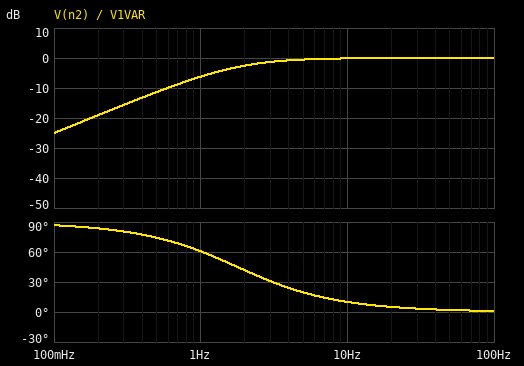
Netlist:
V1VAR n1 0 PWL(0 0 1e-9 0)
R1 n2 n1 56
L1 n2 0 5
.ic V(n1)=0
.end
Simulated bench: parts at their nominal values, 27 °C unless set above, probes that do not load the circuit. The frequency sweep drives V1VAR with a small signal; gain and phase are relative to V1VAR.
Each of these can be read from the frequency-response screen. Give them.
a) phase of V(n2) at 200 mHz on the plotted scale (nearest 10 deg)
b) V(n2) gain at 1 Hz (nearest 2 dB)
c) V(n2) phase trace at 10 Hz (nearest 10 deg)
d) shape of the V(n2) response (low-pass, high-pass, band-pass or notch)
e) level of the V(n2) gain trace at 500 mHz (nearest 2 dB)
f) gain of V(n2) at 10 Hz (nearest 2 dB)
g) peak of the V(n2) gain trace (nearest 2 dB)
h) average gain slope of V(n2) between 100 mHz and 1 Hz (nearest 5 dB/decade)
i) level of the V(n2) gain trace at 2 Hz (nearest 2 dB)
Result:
80 deg
-6 dB
10 deg
high-pass
-12 dB
0 dB
0 dB
20 dB/decade
-2 dB
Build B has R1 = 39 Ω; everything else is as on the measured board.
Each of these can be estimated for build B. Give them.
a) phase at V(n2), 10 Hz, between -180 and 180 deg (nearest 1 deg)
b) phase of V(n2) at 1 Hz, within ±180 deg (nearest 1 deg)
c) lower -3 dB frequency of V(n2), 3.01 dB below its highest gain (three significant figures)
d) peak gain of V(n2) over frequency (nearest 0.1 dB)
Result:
7 deg
51 deg
1.24 Hz
0 dB
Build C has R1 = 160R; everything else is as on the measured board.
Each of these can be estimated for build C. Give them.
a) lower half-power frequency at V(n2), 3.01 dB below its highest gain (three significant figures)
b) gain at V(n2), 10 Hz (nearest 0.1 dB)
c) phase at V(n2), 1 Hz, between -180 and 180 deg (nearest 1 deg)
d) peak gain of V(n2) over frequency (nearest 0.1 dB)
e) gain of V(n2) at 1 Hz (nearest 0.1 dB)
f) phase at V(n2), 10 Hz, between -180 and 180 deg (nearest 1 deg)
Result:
5.09 Hz
-1.0 dB
79 deg
0 dB
-14.3 dB
27 deg
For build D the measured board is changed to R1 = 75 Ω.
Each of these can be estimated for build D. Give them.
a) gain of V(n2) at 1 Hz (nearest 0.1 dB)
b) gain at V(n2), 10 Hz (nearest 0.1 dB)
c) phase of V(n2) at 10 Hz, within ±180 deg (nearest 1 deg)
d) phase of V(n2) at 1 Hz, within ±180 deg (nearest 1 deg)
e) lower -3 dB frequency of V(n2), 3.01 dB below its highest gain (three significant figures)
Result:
-8.3 dB
-0.2 dB
13 deg
67 deg
2.39 Hz
